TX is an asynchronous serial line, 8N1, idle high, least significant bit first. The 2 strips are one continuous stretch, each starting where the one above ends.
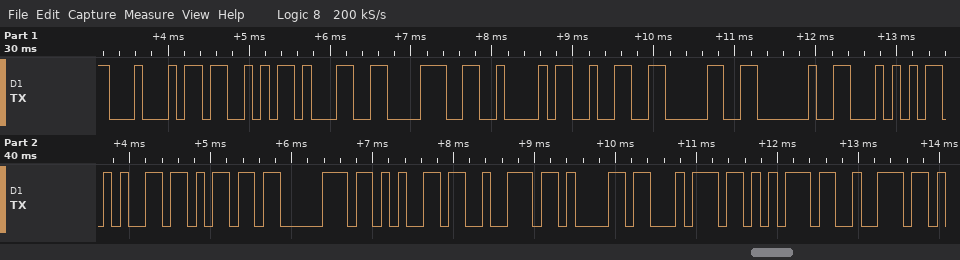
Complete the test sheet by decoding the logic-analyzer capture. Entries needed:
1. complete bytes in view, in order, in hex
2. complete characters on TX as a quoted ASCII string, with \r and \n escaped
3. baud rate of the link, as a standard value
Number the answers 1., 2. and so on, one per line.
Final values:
1. 0x44 0x53 0x31 0x38 0x42 0x32 0x30 0x20 0x54 0x65 0x6D 0x70 0x65 0x72 0x61 0x74 0x75 0x72
2. "DS18B20 Temperatur"
3. 9600 baud
